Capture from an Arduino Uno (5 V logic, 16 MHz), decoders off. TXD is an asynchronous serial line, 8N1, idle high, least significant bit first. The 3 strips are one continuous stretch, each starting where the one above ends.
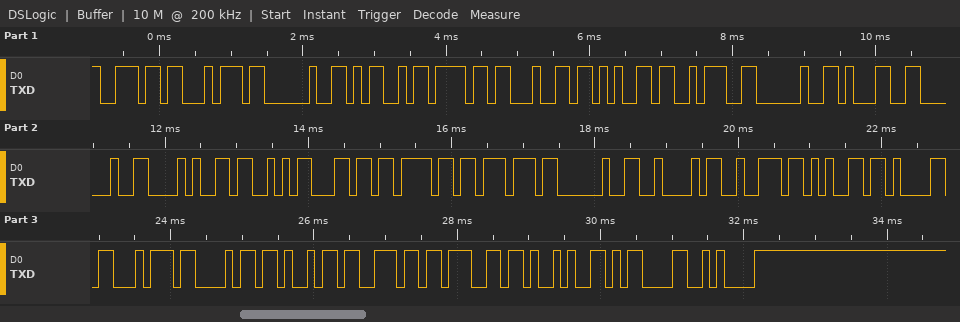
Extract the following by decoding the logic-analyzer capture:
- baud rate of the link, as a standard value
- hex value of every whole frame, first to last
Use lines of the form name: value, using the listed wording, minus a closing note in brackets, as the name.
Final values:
baud rate of the link, as a standard value: 9600 baud
hex value of every whole frame, first to last: 6E 74 20 4D 6F 64 65 3A 20 31 20 28 53 6C 6F 77 20 42 72 65 61 74 68 69 6E 67 29 0D 0A
